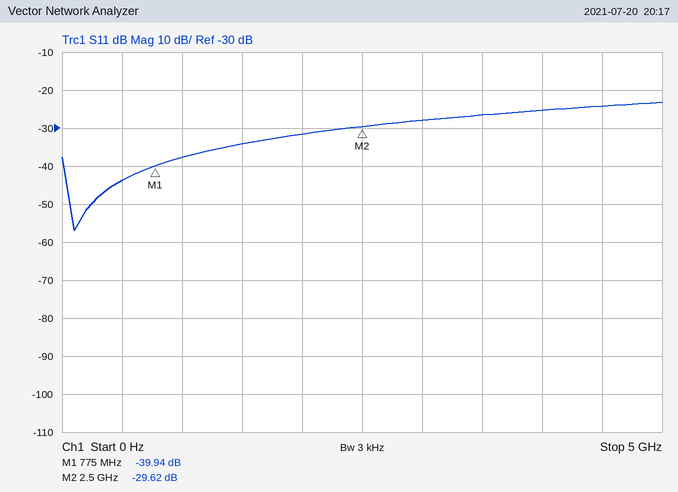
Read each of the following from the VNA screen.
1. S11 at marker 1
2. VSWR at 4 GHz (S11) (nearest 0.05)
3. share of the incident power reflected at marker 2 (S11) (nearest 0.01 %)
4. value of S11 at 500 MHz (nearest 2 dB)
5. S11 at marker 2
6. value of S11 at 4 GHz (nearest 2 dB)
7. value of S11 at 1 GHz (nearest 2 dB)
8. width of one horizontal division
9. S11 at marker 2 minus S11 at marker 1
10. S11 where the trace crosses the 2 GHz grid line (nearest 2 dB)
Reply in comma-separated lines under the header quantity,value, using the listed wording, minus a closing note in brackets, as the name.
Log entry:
quantity,value
S11 at marker 1,-39.94 dB
VSWR at 4 GHz (S11),1.10
share of the incident power reflected at marker 2 (S11),0.11 %
value of S11 at 500 MHz,-44 dB
S11 at marker 2,-29.62 dB
value of S11 at 4 GHz,-26 dB
value of S11 at 1 GHz,-38 dB
width of one horizontal division,500 MHz
S11 at marker 2 minus S11 at marker 1,10.32 dB
S11 where the trace crosses the 2 GHz grid line,-32 dB
